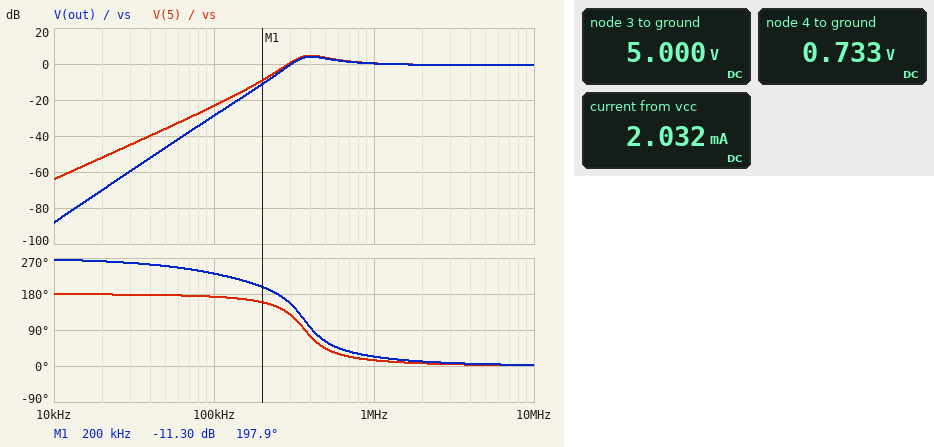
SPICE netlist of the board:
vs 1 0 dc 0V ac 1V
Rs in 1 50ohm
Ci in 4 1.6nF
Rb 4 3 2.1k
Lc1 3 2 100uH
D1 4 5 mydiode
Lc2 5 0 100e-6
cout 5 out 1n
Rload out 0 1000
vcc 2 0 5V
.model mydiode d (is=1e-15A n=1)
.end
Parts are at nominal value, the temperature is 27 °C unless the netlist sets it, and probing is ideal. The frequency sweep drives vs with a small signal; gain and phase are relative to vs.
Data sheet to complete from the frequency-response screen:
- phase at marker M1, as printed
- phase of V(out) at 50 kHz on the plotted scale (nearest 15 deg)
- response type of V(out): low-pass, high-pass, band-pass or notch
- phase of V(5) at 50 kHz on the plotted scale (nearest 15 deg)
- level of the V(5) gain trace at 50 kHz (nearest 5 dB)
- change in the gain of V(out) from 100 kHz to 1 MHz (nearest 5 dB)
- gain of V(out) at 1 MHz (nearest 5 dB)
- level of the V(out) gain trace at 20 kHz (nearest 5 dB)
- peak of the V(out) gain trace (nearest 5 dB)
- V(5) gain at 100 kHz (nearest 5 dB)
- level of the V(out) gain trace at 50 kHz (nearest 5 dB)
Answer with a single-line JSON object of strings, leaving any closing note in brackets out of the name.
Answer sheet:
{"phase at marker M1, as printed": "197.9 deg", "phase of V(out) at 50 kHz on the plotted scale": "255 deg", "response type of V(out): low-pass, high-pass, band-pass or notch": "high-pass", "phase of V(5) at 50 kHz on the plotted scale": "180 deg", "level of the V(5) gain trace at 50 kHz": "-35 dB", "change in the gain of V(out) from 100 kHz to 1 MHz": "30 dB", "gain of V(out) at 1 MHz": "0 dB", "level of the V(out) gain trace at 20 kHz": "-70 dB", "peak of the V(out) gain trace": "5 dB", "V(5) gain at 100 kHz": "-25 dB", "level of the V(out) gain trace at 50 kHz": "-45 dB"}
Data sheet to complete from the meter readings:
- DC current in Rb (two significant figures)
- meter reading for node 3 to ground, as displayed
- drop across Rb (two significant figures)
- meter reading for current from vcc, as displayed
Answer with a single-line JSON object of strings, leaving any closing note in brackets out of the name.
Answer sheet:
{"DC current in Rb": "2.0 mA", "meter reading for node 3 to ground, as displayed": "5.000 V", "drop across Rb": "4.3 V", "meter reading for current from vcc, as displayed": "2.032 mA"}
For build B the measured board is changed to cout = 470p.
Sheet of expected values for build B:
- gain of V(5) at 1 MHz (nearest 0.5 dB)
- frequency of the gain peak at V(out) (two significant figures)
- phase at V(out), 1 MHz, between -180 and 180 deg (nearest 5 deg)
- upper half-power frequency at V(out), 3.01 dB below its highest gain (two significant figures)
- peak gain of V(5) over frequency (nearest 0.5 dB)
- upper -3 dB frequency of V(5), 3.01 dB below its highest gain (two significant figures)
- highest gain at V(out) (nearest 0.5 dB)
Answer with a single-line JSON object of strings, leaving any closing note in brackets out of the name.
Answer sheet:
{"gain of V(5) at 1 MHz": "0.5 dB", "frequency of the gain peak at V(out)": "400 kHz", "phase at V(out), 1 MHz, between -180 and 180 deg": "30 deg", "upper half-power frequency at V(out), 3.01 dB below its highest gain": "730 kHz", "peak gain of V(5) over frequency": "6.0 dB", "upper -3 dB frequency of V(5), 3.01 dB below its highest gain": "550 kHz", "highest gain at V(out)": "3.5 dB"}
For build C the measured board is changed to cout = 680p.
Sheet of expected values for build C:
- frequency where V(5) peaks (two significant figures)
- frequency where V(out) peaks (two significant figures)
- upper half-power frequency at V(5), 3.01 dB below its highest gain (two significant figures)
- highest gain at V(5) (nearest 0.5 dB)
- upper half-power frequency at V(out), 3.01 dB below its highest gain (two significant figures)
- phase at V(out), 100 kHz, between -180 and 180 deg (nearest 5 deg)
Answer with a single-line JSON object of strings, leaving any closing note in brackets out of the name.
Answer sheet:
{"frequency where V(5) peaks": "390 kHz", "frequency where V(out) peaks": "400 kHz", "upper half-power frequency at V(5), 3.01 dB below its highest gain": "610 kHz", "highest gain at V(5)": "5.0 dB", "upper half-power frequency at V(out), 3.01 dB below its highest gain": "730 kHz", "phase at V(out), 100 kHz, between -180 and 180 deg": "-120 deg"}
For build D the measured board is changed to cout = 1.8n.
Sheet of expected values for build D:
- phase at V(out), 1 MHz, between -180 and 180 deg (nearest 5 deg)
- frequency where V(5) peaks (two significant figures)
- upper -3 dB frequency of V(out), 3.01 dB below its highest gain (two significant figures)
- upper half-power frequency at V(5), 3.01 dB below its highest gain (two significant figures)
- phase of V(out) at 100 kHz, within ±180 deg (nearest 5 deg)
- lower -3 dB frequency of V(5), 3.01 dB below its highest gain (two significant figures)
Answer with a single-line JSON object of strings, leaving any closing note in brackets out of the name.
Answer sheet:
{"phase at V(out), 1 MHz, between -180 and 180 deg": "20 deg", "frequency where V(5) peaks": "410 kHz", "upper -3 dB frequency of V(out), 3.01 dB below its highest gain": "760 kHz", "upper half-power frequency at V(5), 3.01 dB below its highest gain": "730 kHz", "phase of V(out) at 100 kHz, within ±180 deg": "-145 deg", "lower -3 dB frequency of V(5), 3.01 dB below its highest gain": "320 kHz"}
